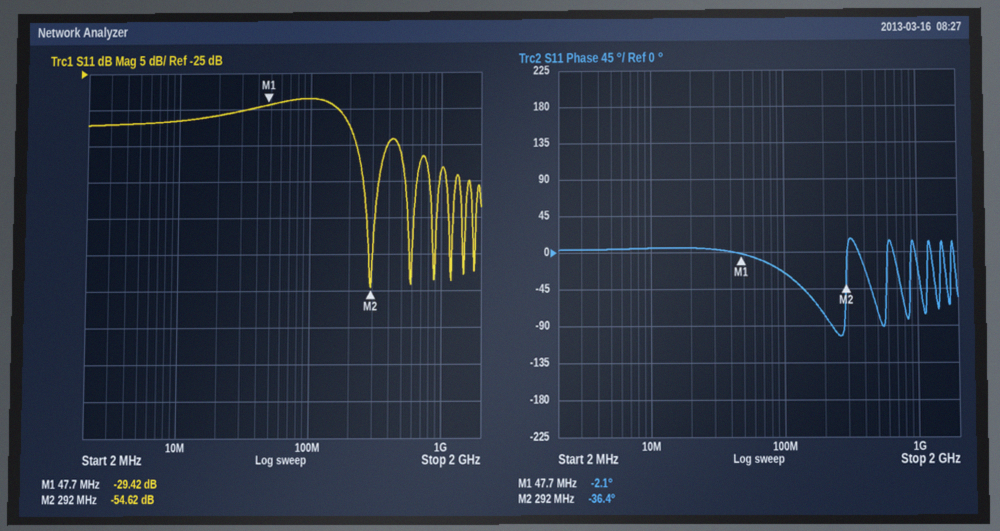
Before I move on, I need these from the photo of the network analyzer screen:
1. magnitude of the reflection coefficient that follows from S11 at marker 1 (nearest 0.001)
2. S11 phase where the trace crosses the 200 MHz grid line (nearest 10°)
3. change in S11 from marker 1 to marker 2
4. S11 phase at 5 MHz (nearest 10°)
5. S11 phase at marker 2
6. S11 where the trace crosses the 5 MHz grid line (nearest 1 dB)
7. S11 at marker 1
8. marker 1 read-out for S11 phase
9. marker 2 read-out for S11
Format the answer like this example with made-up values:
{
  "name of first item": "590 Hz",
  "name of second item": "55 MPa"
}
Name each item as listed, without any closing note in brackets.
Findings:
{
  "magnitude of the reflection coefficient that follows from S11 at marker 1": "0.034",
  "S11 phase where the trace crosses the 200 MHz grid line": "-80°",
  "change in S11 from marker 1 to marker 2": "-25.20 dB",
  "S11 phase at 5 MHz": "0°",
  "S11 phase at marker 2": "-36.4°",
  "S11 where the trace crosses the 5 MHz grid line": "-32 dB",
  "S11 at marker 1": "-29.42 dB",
  "marker 1 read-out for S11 phase": "-2.1°",
  "marker 2 read-out for S11": "-54.62 dB"
}
